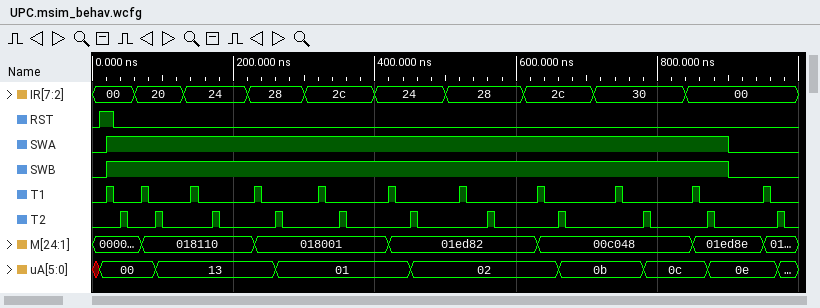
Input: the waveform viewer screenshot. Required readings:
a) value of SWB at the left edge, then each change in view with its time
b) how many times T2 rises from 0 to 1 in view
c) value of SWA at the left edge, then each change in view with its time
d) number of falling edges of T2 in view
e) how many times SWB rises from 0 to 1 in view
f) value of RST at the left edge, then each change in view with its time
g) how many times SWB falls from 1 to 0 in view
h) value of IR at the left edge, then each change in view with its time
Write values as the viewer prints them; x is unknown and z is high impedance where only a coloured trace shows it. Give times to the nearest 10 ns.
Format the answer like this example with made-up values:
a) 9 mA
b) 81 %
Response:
a) 0, 1 at 20 ns, 0 at 900 ns
b) 11
c) 0, 1 at 20 ns, 0 at 900 ns
d) 11
e) 1
f) 0, 1 at 10 ns, 0 at 30 ns
g) 1
h) 00, 20 at 60 ns, 24 at 130 ns, 28 at 220 ns, 2c at 300 ns, 24 at 400 ns, 28 at 500 ns, 2c at 610 ns, 30 at 710 ns, 00 at 840 ns
